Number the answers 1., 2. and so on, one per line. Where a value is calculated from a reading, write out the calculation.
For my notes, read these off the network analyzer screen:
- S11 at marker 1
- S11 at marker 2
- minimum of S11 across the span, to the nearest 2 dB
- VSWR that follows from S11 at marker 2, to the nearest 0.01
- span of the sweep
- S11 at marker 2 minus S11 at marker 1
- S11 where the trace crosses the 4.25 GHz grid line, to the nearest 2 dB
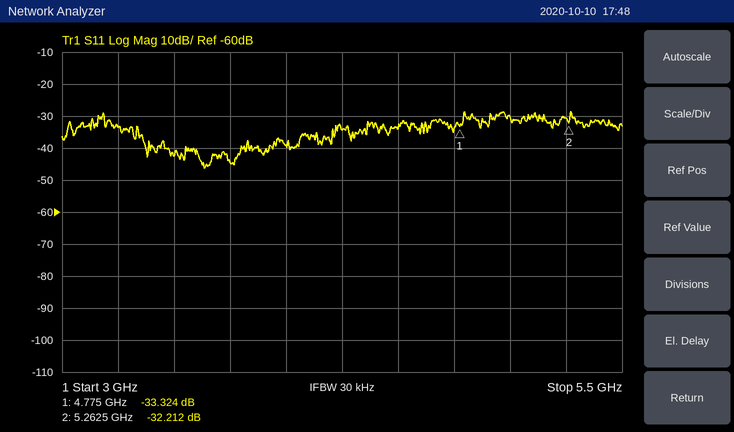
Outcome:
1. -33.324 dB
2. -32.212 dB
3. -46 dB
4. (1 + 0.0245)/(1 − 0.0245) ≈ 1.05
5. 2.5 GHz
6. -32.212 − (-33.324) = 1.112 dB
7. -34 dB
